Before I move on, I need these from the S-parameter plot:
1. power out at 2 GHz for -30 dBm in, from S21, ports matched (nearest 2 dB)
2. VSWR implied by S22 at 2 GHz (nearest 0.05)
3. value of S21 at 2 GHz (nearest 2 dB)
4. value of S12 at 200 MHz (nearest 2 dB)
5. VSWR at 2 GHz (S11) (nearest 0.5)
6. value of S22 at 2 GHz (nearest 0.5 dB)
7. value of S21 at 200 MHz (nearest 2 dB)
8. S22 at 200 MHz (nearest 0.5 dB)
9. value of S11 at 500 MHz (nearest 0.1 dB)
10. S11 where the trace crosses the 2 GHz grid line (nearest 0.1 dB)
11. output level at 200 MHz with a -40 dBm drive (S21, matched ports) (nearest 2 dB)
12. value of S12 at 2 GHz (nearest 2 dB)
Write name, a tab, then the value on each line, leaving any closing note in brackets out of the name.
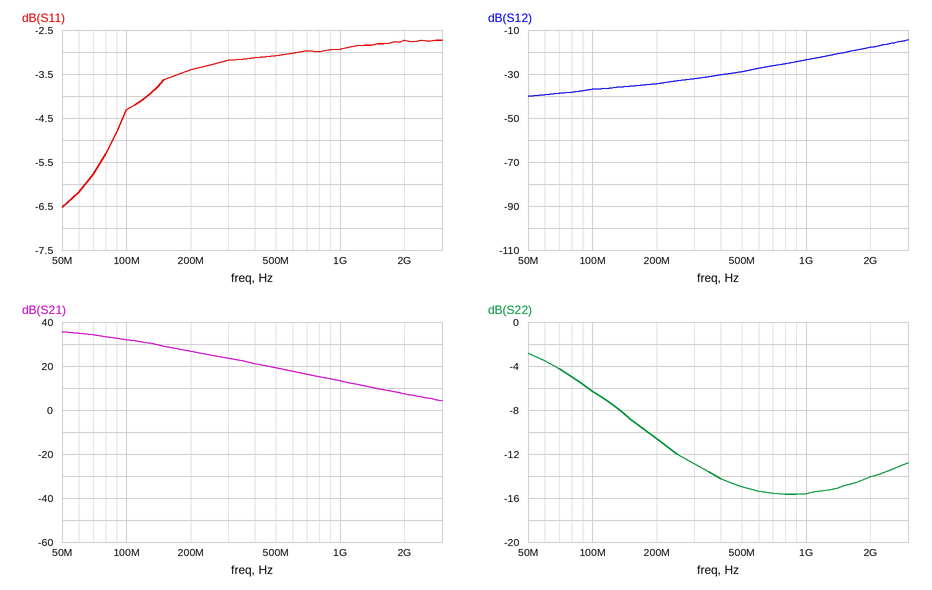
power out at 2 GHz for -30 dBm in, from S21, ports matched	-22 dBm
VSWR implied by S22 at 2 GHz	1.50
value of S21 at 2 GHz	8 dB
value of S12 at 200 MHz	-34 dB
VSWR at 2 GHz (S11)	6.5
value of S22 at 2 GHz	-14.0 dB
value of S21 at 200 MHz	26 dB
S22 at 200 MHz	-10.5 dB
value of S11 at 500 MHz	-3.1 dB
S11 where the trace crosses the 2 GHz grid line	-2.7 dB
output level at 200 MHz with a -40 dBm drive (S21, matched ports)	-14 dBm
value of S12 at 2 GHz	-18 dB
